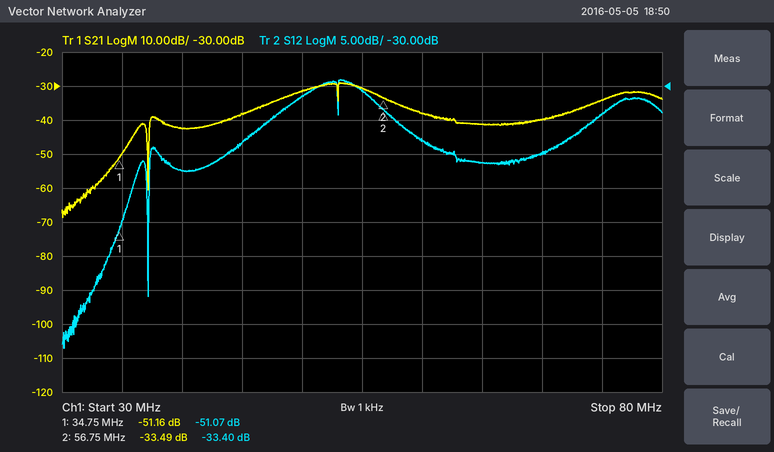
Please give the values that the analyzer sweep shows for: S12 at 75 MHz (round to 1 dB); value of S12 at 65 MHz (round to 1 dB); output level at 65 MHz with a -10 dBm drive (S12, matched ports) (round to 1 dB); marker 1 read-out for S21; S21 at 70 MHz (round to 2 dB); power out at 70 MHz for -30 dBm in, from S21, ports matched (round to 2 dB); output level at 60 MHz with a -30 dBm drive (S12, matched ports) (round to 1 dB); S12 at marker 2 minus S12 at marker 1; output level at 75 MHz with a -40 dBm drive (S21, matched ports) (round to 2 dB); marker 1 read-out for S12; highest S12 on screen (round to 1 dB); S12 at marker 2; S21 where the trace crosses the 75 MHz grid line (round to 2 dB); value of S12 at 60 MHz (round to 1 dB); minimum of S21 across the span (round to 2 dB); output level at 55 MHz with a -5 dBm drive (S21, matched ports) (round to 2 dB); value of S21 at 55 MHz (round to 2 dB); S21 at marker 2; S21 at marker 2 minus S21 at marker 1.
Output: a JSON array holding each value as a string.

["-34 dB", "-41 dB", "-51 dBm", "-51.16 dB", "-40 dB", "-70 dBm", "-68 dBm", "17.67 dB", "-74 dBm", "-51.07 dB", "-29 dB", "-33.40 dB", "-34 dB", "-38 dB", "-68 dB", "-36 dBm", "-30 dB", "-33.49 dB", "17.67 dB"]
